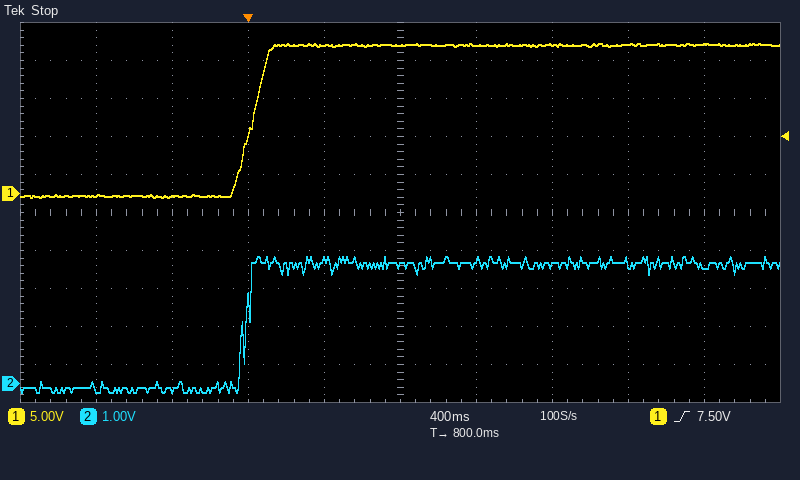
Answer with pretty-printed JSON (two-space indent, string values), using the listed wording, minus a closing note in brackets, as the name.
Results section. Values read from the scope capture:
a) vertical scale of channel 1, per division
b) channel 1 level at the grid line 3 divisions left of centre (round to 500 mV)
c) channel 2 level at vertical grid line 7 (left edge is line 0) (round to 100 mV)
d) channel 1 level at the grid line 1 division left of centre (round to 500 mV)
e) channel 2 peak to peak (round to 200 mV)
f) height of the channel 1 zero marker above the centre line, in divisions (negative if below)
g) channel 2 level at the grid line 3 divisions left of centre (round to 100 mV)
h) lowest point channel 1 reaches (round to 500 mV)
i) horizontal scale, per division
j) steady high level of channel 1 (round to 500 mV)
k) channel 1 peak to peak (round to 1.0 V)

{
  "vertical scale of channel 1, per division": "5 V",
  "channel 1 level at the grid line 3 divisions left of centre": "-500 mV",
  "channel 2 level at vertical grid line 7 (left edge is line 0)": "3.1 V",
  "channel 1 level at the grid line 1 division left of centre": "19.5 V",
  "channel 2 peak to peak": "3.6 V",
  "height of the channel 1 zero marker above the centre line, in divisions": "+0.5 div",
  "channel 2 level at the grid line 3 divisions left of centre": "-200 mV",
  "lowest point channel 1 reaches": "-500 mV",
  "horizontal scale, per division": "400 ms",
  "steady high level of channel 1": "19.5 V",
  "channel 1 peak to peak": "20.0 V"
}
